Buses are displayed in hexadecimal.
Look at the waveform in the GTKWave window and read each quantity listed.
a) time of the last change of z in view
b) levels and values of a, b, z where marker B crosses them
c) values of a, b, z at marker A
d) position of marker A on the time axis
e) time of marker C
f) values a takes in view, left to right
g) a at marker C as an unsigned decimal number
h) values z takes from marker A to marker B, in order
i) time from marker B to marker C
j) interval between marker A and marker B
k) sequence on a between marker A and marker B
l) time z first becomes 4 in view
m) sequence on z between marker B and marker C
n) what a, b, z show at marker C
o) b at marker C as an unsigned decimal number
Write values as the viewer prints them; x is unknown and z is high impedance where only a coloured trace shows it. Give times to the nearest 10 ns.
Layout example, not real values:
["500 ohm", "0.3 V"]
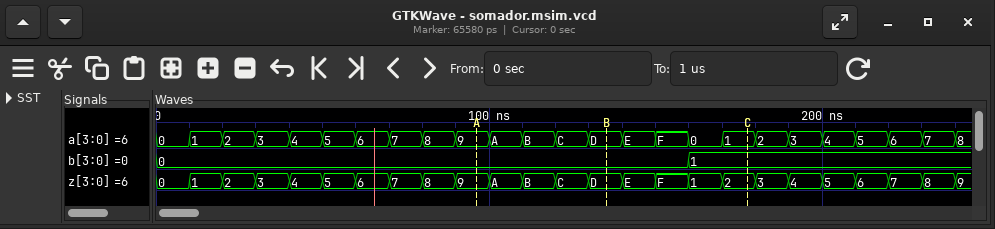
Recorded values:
["240 ns", "a=D, b=0, z=D", "a=9, b=0, z=9", "100 ns", "180 ns", "0, 1, 2, 3, 4, 5, 6, 7, 8, 9, A, B, C, D, E, F, 0, 1, 2, 3, 4, 5, 6, 7, 8", "1", "9, A, B, C, D", "40 ns", "40 ns", "9, A, B, C, D", "40 ns", "D, E, F, 1, 2", "a=1, b=1, z=2", "1"]
